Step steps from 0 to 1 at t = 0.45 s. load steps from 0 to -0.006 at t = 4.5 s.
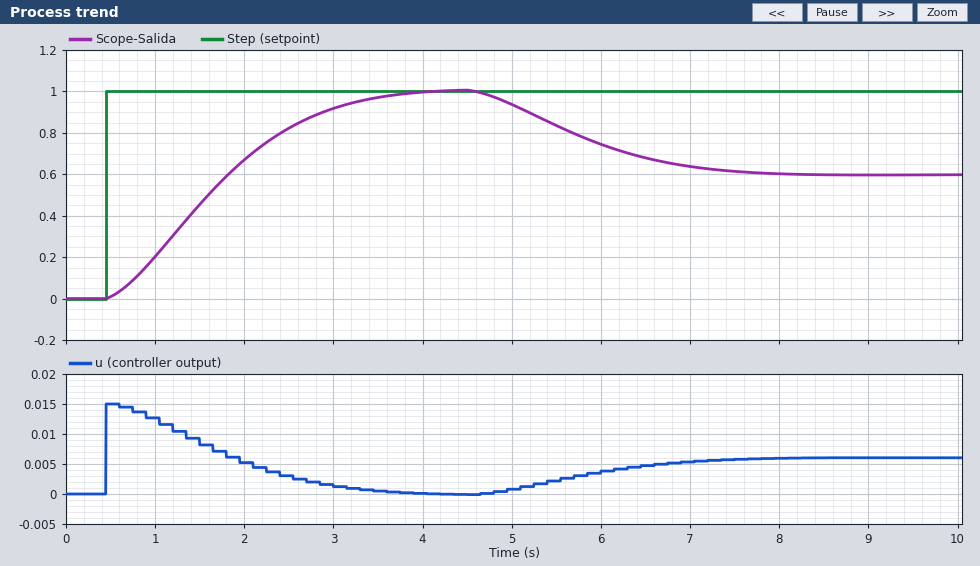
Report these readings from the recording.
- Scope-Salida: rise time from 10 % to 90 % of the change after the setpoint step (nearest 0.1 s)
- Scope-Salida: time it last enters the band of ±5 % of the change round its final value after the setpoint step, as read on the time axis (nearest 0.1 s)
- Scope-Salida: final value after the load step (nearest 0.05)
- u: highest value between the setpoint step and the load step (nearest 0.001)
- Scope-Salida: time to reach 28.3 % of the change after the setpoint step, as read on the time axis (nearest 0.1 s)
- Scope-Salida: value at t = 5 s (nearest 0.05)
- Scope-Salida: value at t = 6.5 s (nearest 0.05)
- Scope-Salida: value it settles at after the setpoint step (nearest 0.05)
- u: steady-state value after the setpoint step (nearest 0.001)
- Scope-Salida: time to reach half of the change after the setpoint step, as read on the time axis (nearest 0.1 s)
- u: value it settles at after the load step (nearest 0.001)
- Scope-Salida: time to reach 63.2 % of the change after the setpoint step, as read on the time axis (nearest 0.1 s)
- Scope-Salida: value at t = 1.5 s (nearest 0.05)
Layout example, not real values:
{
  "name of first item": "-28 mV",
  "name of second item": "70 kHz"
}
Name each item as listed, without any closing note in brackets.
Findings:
{
  "Scope-Salida: rise time from 10 % to 90 % of the change after the setpoint step": "2.1 s",
  "Scope-Salida: time it last enters the band of ±5 % of the change round its final value after the setpoint step, as read on the time axis": "3.3 s",
  "Scope-Salida: final value after the load step": "0.60",
  "u: highest value between the setpoint step and the load step": "0.015",
  "Scope-Salida: time to reach 28.3 % of the change after the setpoint step, as read on the time axis": "1.2 s",
  "Scope-Salida: value at t = 5 s": "0.95",
  "Scope-Salida: value at t = 6.5 s": "0.70",
  "Scope-Salida: value it settles at after the setpoint step": "1.00",
  "u: steady-state value after the setpoint step": "0.000",
  "Scope-Salida: time to reach half of the change after the setpoint step, as read on the time axis": "1.6 s",
  "u: value it settles at after the load step": "0.006",
  "Scope-Salida: time to reach 63.2 % of the change after the setpoint step, as read on the time axis": "1.9 s",
  "Scope-Salida: value at t = 1.5 s": "0.45"
}
